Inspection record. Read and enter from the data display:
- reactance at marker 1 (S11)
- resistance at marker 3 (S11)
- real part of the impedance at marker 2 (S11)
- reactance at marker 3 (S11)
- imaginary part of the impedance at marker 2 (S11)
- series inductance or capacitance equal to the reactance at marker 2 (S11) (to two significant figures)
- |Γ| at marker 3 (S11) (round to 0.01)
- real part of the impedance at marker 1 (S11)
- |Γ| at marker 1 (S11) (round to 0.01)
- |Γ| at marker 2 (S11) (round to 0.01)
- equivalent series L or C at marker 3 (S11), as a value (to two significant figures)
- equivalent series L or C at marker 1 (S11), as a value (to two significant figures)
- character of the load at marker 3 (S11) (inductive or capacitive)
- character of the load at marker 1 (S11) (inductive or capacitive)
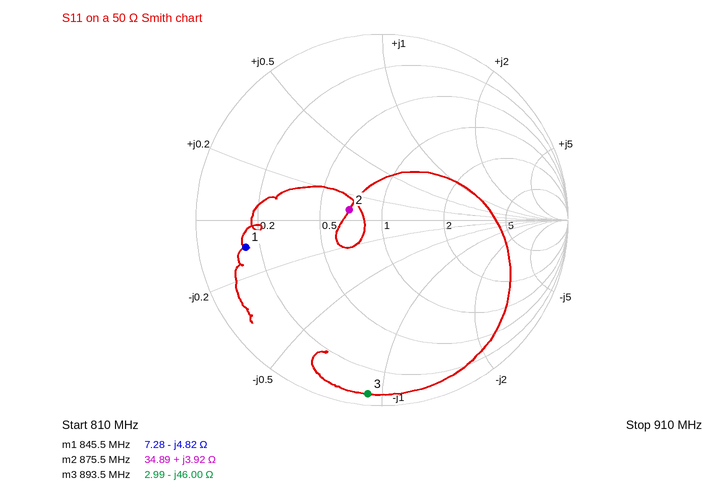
-4.82 Ω
2.99 Ω
34.89 Ω
-46.00 Ω
+3.92 Ω
710 pH
0.94
7.28 Ω
0.75
0.18
3.9 pF
39 pF
capacitive
capacitive
